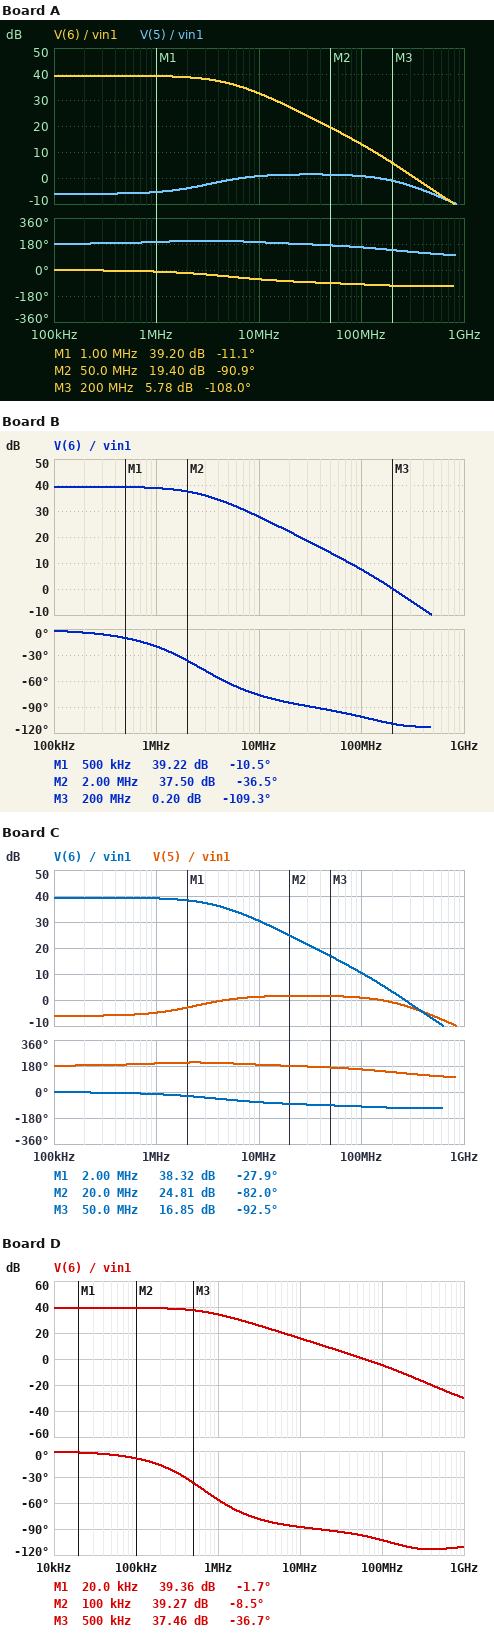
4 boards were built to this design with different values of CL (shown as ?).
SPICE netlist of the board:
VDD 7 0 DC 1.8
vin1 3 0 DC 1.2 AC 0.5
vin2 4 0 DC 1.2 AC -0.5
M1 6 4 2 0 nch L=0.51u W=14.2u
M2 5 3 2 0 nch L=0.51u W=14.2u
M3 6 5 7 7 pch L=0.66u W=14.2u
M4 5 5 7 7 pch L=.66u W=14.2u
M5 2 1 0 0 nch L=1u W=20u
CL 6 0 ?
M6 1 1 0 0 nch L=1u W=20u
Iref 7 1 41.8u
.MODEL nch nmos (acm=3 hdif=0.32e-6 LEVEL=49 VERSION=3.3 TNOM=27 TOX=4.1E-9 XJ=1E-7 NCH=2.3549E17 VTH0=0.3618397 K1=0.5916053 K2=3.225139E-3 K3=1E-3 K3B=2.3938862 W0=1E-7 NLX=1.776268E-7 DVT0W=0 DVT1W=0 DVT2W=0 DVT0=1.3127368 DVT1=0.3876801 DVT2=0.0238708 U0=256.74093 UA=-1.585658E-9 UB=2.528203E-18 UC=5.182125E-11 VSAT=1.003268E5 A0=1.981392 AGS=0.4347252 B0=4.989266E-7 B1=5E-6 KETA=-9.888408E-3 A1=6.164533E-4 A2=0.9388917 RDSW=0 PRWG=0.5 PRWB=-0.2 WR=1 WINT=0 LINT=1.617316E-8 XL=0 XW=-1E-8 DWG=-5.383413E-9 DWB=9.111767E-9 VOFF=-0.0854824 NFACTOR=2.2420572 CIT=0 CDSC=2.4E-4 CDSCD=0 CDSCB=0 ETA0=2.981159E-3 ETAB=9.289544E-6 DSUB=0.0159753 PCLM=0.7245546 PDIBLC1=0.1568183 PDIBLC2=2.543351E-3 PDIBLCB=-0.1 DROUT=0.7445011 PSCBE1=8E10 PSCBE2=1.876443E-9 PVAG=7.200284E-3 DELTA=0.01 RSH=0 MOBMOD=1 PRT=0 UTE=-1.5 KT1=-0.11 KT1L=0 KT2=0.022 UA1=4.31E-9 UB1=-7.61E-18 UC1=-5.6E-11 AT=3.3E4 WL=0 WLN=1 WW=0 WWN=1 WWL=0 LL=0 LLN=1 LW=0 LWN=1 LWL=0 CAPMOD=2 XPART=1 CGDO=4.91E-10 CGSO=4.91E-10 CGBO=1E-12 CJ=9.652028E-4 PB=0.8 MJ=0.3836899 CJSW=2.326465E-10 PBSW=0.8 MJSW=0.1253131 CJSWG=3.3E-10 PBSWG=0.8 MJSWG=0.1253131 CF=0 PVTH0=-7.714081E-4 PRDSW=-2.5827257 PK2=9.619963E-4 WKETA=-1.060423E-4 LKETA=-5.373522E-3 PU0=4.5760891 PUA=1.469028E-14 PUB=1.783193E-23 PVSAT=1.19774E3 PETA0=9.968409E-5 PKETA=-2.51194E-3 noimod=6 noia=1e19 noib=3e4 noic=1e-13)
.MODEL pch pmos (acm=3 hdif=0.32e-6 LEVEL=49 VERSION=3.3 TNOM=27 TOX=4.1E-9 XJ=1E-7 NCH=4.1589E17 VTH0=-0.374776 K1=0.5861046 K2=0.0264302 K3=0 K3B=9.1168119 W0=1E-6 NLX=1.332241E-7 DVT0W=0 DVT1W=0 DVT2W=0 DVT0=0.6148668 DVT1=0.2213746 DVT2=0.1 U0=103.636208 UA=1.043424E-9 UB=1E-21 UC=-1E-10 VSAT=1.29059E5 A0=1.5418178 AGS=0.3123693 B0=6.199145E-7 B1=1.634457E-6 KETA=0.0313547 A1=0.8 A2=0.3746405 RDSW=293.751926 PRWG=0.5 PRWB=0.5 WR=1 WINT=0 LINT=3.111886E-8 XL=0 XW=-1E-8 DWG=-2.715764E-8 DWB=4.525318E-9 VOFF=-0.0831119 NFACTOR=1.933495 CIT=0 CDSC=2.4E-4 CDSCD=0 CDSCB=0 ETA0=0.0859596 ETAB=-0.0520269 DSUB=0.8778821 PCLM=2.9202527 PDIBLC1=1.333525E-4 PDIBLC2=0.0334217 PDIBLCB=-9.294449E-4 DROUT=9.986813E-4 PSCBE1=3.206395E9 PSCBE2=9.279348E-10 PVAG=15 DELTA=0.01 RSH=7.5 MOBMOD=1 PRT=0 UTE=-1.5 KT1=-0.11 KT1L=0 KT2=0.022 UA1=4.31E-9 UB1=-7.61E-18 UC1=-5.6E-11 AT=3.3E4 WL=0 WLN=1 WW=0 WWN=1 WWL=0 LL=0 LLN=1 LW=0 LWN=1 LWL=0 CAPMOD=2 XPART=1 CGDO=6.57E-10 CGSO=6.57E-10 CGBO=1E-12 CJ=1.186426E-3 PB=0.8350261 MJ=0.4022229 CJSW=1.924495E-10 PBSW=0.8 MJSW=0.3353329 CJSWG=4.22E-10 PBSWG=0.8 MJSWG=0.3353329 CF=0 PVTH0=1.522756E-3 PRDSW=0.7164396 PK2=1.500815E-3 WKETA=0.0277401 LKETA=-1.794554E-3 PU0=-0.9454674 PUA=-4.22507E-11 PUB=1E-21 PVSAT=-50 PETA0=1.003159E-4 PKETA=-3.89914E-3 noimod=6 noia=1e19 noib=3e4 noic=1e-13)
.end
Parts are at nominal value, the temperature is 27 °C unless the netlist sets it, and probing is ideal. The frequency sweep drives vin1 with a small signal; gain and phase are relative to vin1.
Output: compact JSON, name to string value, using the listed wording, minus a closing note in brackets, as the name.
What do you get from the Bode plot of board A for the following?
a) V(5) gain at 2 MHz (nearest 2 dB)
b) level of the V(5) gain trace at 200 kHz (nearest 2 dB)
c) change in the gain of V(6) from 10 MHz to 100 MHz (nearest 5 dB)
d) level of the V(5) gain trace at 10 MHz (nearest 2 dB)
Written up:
{"V(5) gain at 2 MHz": "-4 dB", "level of the V(5) gain trace at 200 kHz": "-6 dB", "change in the gain of V(6) from 10 MHz to 100 MHz": "-20 dB", "level of the V(5) gain trace at 10 MHz": "0 dB"}
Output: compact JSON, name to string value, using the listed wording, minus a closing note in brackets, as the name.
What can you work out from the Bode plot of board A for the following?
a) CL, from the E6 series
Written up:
{"CL, from the E6 series": "150 fF"}
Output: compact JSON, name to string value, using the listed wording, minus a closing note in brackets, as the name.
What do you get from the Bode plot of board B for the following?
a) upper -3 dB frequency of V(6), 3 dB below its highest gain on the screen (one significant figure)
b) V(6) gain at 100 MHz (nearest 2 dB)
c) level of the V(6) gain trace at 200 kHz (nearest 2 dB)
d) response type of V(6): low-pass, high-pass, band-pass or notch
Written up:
{"upper -3 dB frequency of V(6), 3 dB below its highest gain on the screen": "3 MHz", "V(6) gain at 100 MHz": "8 dB", "level of the V(6) gain trace at 200 kHz": "40 dB", "response type of V(6): low-pass, high-pass, band-pass or notch": "low-pass"}
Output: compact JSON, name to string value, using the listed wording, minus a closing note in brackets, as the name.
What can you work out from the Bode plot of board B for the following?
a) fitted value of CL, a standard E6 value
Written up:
{"fitted value of CL, a standard E6 value": "330 fF"}
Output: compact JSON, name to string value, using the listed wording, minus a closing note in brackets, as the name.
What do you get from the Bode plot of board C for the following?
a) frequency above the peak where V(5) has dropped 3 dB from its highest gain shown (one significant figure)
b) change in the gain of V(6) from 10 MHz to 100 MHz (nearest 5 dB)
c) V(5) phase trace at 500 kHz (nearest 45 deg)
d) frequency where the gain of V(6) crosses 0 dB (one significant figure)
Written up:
{"frequency above the peak where V(5) has dropped 3 dB from its highest gain shown": "200 MHz", "change in the gain of V(6) from 10 MHz to 100 MHz": "-20 dB", "V(5) phase trace at 500 kHz": "180 deg", "frequency where the gain of V(6) crosses 0 dB": "300 MHz"}
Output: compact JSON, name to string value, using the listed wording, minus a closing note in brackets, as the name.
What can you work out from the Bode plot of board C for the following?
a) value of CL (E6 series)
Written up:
{"value of CL": "220 fF"}
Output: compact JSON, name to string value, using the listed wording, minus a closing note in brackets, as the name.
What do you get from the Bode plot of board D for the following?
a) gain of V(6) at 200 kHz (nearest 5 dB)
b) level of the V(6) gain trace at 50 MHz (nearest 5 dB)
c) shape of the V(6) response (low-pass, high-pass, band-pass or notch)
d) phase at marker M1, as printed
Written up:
{"gain of V(6) at 200 kHz": "40 dB", "level of the V(6) gain trace at 50 MHz": "0 dB", "shape of the V(6) response": "low-pass", "phase at marker M1, as printed": "-1.7 deg"}
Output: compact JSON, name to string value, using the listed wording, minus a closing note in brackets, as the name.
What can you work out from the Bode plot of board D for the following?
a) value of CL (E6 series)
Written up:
{"value of CL": "1.5 pF"}
